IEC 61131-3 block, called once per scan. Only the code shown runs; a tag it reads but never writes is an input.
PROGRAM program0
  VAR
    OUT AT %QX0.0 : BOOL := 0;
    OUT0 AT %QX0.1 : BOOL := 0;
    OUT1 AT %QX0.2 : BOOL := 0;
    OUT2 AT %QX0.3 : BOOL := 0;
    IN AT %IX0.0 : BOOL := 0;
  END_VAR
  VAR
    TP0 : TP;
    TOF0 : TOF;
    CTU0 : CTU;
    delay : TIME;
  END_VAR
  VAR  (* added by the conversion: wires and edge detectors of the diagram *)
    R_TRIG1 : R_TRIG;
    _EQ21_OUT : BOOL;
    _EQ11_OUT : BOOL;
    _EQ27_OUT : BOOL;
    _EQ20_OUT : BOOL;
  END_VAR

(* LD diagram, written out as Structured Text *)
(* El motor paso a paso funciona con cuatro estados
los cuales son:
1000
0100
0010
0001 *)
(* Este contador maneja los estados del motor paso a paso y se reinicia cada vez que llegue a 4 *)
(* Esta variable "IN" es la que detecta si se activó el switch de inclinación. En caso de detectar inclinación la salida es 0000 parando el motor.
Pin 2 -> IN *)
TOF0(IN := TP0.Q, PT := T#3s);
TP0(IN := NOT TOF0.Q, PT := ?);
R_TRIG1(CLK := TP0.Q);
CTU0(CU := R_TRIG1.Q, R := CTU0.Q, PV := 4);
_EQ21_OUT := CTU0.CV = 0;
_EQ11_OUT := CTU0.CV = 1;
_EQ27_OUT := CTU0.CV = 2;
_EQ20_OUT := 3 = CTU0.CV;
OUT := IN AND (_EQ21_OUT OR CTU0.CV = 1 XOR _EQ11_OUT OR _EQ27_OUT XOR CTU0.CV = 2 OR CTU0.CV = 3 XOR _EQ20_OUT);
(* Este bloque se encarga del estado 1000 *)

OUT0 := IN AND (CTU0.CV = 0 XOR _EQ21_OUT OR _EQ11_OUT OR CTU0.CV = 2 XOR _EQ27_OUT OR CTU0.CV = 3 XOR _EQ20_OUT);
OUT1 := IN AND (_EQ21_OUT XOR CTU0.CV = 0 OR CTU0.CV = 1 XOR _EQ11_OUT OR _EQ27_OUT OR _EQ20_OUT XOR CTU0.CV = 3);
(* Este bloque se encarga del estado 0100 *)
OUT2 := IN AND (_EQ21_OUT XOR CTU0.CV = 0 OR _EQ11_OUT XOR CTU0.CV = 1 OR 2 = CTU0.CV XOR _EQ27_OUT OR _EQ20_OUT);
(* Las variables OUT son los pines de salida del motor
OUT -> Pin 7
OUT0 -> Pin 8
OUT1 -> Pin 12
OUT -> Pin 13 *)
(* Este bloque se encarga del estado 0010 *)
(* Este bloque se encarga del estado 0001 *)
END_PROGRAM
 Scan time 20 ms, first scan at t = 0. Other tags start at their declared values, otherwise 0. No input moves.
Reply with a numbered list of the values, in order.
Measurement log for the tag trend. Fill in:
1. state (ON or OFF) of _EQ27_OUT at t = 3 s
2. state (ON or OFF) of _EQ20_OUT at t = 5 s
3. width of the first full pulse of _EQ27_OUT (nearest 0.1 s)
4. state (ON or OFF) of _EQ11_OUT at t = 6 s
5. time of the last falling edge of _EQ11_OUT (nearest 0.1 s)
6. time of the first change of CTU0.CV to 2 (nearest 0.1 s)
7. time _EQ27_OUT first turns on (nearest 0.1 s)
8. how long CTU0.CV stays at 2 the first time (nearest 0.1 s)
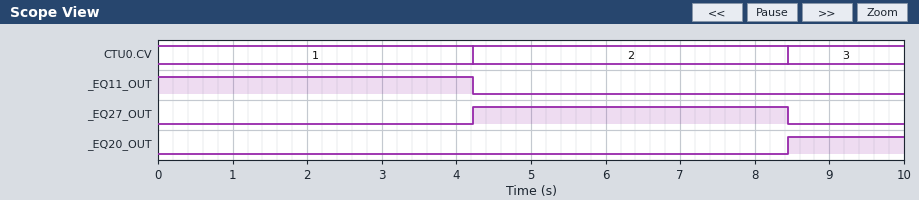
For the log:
1. OFF
2. OFF
3. 4.2 s
4. OFF
5. 4.2 s
6. 4.2 s
7. 4.2 s
8. 4.2 s
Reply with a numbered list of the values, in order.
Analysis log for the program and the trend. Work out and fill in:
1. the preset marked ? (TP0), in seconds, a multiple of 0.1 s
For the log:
1. 1.2 s
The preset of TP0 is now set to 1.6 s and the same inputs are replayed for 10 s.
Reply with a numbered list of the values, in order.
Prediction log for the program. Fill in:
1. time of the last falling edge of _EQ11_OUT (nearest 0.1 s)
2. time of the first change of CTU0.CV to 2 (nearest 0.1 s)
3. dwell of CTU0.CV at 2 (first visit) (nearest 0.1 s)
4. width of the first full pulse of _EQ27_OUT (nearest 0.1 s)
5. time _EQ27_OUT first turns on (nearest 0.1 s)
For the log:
1. 4.6 s
2. 4.6 s
3. 4.6 s
4. 4.6 s
5. 4.6 s
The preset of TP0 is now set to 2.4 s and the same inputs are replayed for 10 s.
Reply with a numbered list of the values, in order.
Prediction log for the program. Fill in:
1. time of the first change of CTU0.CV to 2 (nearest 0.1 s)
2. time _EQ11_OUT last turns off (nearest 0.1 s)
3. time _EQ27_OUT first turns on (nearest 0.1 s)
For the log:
1. 5.4 s
2. 5.4 s
3. 5.4 s
